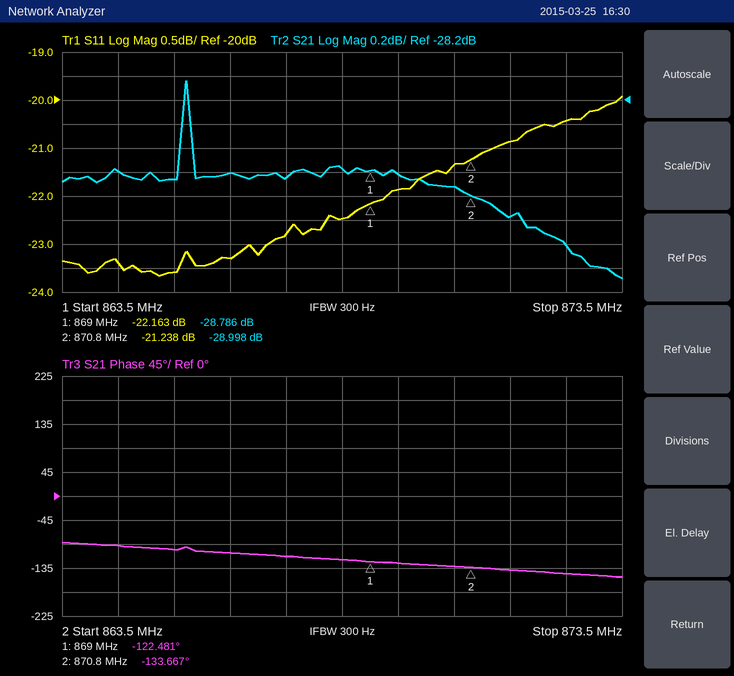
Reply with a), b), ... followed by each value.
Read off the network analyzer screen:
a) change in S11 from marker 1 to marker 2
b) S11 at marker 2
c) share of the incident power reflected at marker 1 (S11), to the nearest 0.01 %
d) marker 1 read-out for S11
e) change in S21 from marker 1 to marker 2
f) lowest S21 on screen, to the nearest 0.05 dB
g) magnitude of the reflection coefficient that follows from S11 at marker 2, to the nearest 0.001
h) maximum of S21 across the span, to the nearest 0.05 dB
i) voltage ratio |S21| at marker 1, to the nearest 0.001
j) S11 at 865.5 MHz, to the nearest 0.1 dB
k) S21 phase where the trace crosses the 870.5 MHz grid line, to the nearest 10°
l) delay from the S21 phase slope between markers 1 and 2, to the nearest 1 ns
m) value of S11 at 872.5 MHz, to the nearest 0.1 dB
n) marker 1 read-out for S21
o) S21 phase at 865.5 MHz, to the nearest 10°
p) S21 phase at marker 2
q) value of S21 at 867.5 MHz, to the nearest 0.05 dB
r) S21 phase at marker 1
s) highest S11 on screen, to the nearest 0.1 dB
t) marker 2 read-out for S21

a) 0.925 dB
b) -21.238 dB
c) 0.61 %
d) -22.163 dB
e) -0.212 dB
f) -29.70 dB
g) 0.087
h) -28.05 dB
i) 0.036
j) -23.6 dB
k) -130°
l) 17 ns
m) -20.4 dB
n) -28.786 dB
o) -100°
p) -133.667°
q) -28.85 dB
r) -122.481°
s) -19.9 dB
t) -28.998 dB
